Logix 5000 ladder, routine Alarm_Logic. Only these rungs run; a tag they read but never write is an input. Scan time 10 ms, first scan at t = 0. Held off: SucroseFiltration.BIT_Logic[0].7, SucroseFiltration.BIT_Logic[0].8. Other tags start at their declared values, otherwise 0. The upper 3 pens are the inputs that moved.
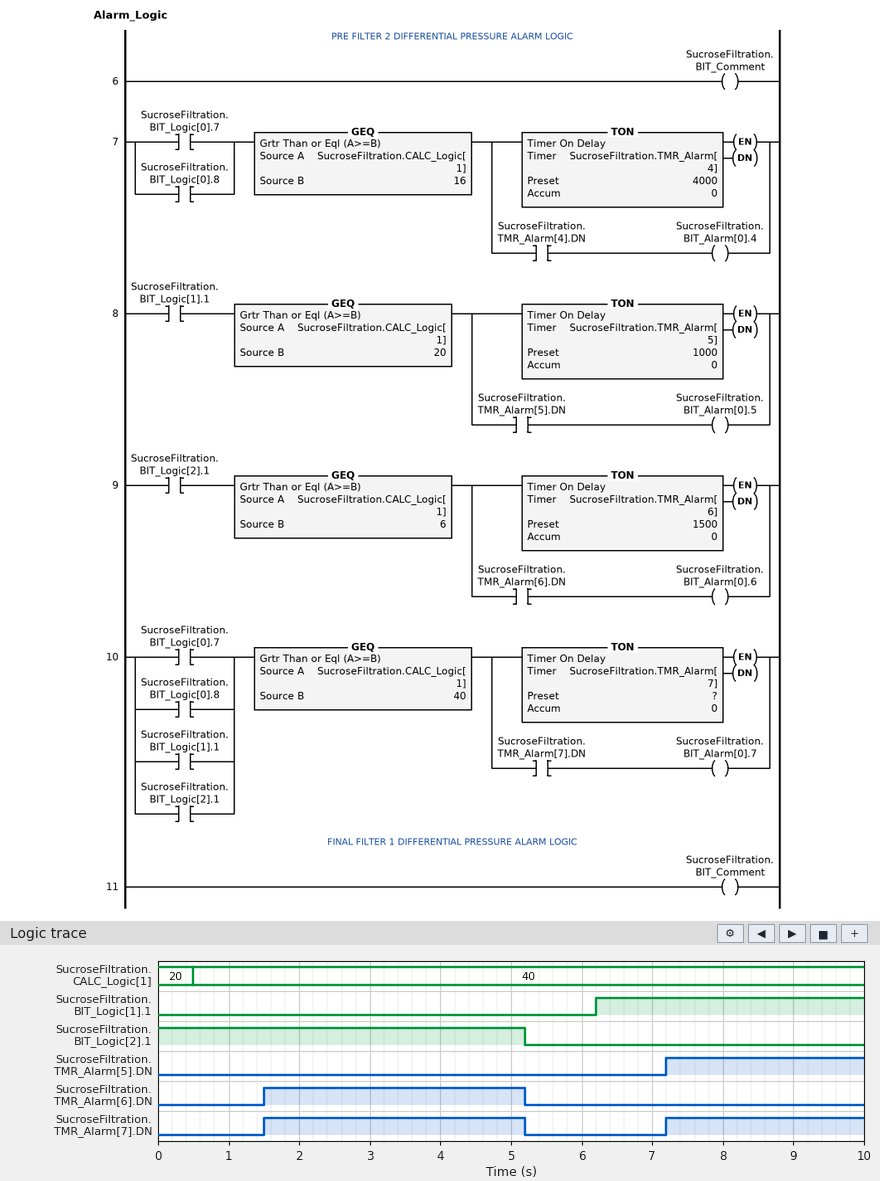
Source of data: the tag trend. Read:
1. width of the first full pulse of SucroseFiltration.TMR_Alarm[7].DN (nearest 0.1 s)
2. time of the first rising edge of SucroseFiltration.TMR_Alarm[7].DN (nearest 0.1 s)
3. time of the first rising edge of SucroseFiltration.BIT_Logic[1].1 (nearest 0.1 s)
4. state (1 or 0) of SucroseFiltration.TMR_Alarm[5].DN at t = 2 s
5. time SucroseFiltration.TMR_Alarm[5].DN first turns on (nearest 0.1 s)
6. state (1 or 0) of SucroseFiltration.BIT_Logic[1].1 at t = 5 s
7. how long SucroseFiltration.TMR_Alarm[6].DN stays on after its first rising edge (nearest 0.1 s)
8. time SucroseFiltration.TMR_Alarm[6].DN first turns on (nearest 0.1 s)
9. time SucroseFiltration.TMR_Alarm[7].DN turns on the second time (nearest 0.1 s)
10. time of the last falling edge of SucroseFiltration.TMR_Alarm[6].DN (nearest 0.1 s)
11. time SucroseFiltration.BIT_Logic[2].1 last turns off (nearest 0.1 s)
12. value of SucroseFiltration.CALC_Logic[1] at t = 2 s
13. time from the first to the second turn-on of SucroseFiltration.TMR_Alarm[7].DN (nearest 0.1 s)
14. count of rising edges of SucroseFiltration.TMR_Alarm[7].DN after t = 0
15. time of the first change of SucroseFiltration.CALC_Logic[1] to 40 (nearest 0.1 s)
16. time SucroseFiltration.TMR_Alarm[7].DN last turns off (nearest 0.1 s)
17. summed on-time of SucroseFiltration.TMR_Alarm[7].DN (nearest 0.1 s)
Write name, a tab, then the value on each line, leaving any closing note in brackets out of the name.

width of the first full pulse of SucroseFiltration.TMR_Alarm[7].DN	3.7 s
time of the first rising edge of SucroseFiltration.TMR_Alarm[7].DN	1.5 s
time of the first rising edge of SucroseFiltration.BIT_Logic[1].1	6.2 s
state (1 or 0) of SucroseFiltration.TMR_Alarm[5].DN at t = 2 s	0
time SucroseFiltration.TMR_Alarm[5].DN first turns on	7.2 s
state (1 or 0) of SucroseFiltration.BIT_Logic[1].1 at t = 5 s	0
how long SucroseFiltration.TMR_Alarm[6].DN stays on after its first rising edge	3.7 s
time SucroseFiltration.TMR_Alarm[6].DN first turns on	1.5 s
time SucroseFiltration.TMR_Alarm[7].DN turns on the second time	7.2 s
time of the last falling edge of SucroseFiltration.TMR_Alarm[6].DN	5.2 s
time SucroseFiltration.BIT_Logic[2].1 last turns off	5.2 s
value of SucroseFiltration.CALC_Logic[1] at t = 2 s	40
time from the first to the second turn-on of SucroseFiltration.TMR_Alarm[7].DN	5.7 s
count of rising edges of SucroseFiltration.TMR_Alarm[7].DN after t = 0	2
time of the first change of SucroseFiltration.CALC_Logic[1] to 40	0.5 s
time SucroseFiltration.TMR_Alarm[7].DN last turns off	5.2 s
summed on-time of SucroseFiltration.TMR_Alarm[7].DN	6.5 s
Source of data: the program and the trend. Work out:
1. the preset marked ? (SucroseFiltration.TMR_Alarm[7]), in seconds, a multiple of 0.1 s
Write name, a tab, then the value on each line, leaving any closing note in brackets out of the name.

the preset marked ? (SucroseFiltration.TMR_Alarm[7]), in seconds, a multiple of 0.1 s	1.0 s
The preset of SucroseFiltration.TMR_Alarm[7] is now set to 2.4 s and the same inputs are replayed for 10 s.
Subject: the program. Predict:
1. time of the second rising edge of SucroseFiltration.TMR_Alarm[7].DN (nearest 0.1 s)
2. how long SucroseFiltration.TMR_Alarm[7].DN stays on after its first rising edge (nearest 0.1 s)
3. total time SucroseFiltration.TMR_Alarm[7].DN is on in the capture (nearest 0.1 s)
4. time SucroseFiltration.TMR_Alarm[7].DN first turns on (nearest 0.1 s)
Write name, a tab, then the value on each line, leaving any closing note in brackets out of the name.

time of the second rising edge of SucroseFiltration.TMR_Alarm[7].DN	8.6 s
how long SucroseFiltration.TMR_Alarm[7].DN stays on after its first rising edge	2.3 s
total time SucroseFiltration.TMR_Alarm[7].DN is on in the capture	3.7 s
time SucroseFiltration.TMR_Alarm[7].DN first turns on	2.9 s
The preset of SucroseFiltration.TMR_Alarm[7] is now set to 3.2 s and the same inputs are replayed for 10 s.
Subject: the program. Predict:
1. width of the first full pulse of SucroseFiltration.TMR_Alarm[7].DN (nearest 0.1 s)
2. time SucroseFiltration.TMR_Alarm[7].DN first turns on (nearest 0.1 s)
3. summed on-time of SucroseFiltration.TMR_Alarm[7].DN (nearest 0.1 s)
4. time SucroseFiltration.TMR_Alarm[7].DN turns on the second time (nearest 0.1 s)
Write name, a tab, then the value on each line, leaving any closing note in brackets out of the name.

width of the first full pulse of SucroseFiltration.TMR_Alarm[7].DN	1.5 s
time SucroseFiltration.TMR_Alarm[7].DN first turns on	3.7 s
summed on-time of SucroseFiltration.TMR_Alarm[7].DN	2.1 s
time SucroseFiltration.TMR_Alarm[7].DN turns on the second time	9.4 s
